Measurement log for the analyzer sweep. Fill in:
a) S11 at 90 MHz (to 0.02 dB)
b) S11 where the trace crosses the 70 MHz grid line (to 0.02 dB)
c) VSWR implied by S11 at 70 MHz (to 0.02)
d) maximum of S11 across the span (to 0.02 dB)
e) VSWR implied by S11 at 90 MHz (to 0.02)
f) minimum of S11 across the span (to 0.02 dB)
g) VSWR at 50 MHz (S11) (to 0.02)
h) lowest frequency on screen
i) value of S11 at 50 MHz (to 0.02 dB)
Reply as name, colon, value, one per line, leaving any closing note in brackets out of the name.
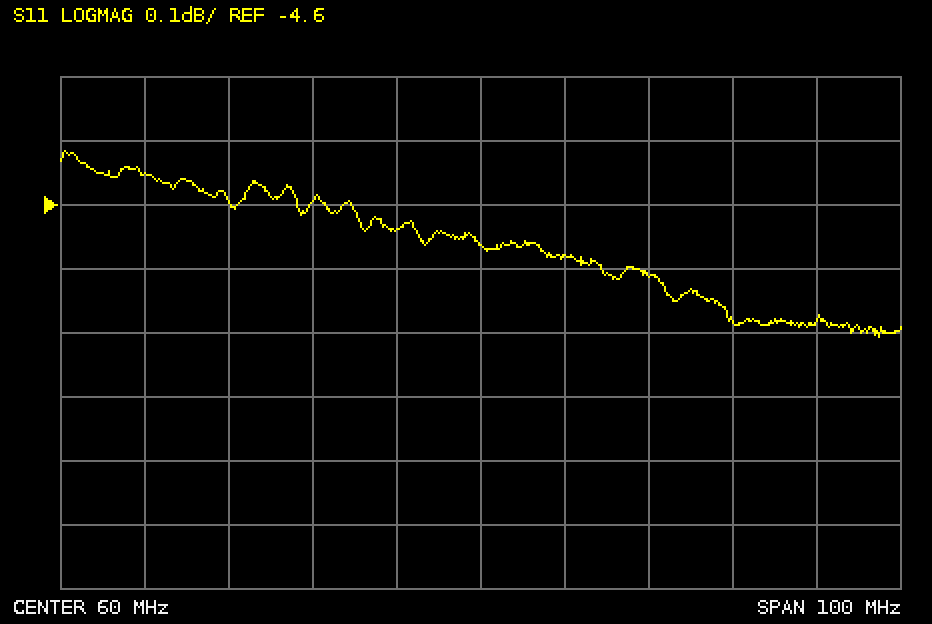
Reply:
S11 at 90 MHz: -4.78 dB
S11 where the trace crosses the 70 MHz grid line: -4.68 dB
VSWR implied by S11 at 70 MHz: 3.80
maximum of S11 across the span: -4.52 dB
VSWR implied by S11 at 90 MHz: 3.72
minimum of S11 across the span: -4.80 dB
VSWR at 50 MHz (S11): 3.84
lowest frequency on screen: 10 MHz
value of S11 at 50 MHz: -4.64 dB
